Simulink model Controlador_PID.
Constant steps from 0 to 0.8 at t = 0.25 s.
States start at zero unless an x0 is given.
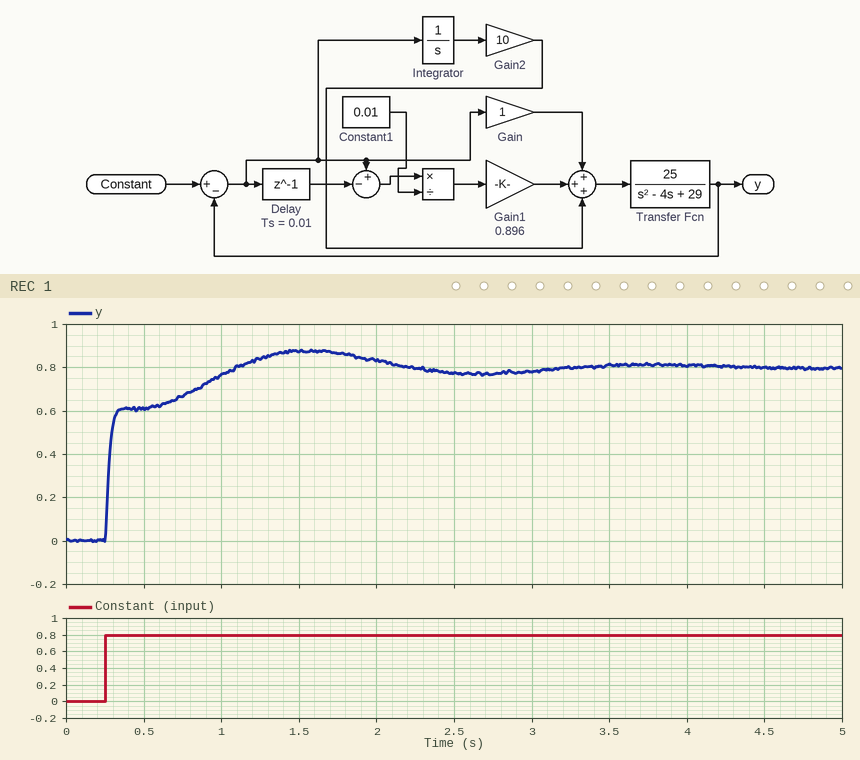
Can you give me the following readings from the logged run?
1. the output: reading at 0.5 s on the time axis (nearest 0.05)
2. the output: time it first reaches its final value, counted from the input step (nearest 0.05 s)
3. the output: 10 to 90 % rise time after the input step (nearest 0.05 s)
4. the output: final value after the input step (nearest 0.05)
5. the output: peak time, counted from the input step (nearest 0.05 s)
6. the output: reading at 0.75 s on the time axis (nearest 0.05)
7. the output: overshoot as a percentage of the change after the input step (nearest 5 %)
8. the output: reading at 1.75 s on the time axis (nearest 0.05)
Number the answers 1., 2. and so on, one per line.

1. 0.60
2. 0.85 s
3. 0.65 s
4. 0.80
5. 1.30 s
6. 0.65
7. 10 %
8. 0.85
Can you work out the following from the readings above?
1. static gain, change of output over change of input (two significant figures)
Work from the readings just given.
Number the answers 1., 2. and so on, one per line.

1. 1.0
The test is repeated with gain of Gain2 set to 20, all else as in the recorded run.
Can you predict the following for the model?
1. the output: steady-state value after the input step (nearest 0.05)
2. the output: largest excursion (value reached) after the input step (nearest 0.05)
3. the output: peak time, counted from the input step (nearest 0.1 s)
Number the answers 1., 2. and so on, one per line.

1. 0.80
2. 0.90
3. 0.8 s
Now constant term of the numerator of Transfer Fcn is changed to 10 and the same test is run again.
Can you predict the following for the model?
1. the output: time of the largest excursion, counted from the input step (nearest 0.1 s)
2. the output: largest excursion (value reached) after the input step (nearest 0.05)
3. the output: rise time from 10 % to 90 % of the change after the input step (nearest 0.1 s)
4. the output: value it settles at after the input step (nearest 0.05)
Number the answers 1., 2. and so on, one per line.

1. 1.5 s
2. 0.85
3. 1.0 s
4. 0.80
